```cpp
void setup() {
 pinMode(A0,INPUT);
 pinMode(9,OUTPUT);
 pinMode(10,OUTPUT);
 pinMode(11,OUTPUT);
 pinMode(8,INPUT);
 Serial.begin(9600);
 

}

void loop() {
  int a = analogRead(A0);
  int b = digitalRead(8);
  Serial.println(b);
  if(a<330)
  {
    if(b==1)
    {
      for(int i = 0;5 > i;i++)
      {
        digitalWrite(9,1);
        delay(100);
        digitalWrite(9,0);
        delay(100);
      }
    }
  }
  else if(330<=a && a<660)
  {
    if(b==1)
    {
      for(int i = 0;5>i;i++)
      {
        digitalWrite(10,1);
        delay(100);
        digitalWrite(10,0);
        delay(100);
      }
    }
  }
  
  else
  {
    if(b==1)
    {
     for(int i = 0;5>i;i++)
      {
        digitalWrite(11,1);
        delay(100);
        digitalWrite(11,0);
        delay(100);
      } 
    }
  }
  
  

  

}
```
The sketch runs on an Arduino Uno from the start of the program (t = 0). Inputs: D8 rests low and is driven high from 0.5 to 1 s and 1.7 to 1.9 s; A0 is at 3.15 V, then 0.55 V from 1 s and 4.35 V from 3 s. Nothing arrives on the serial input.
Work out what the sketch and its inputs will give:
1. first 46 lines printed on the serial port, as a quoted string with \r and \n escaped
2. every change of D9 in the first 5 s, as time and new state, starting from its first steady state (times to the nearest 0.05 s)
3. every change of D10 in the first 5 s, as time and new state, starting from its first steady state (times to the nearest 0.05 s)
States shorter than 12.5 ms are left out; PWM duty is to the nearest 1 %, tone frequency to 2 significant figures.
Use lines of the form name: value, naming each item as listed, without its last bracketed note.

first 46 lines printed on the serial port, as a quoted string with \r and \n escaped: "0\r\n0\r\n0\r\n0\r\n0\r\n0\r\n0\r\n0\r\n0\r\n0\r\n0\r\n0\r\n0\r\n0\r\n0\r\n0\r\n0\r\n0\r\n0\r\n0\r\n0\r\n0\r\n0\r\n0\r\n0\r\n0\r\n0\r\n0\r\n0\r\n0\r\n0\r\n0\r\n0\r\n0\r\n0\r\n0\r\n0\r\n0\r\n0\r\n0\r\n0\r\n0\r\n0\r\n0\r\n0\r\n0\r\n"
every change of D9 in the first 5 s, as time and new state, starting from its first steady state: 0 s low; 1.7 s high; 1.8 s low; 1.9 s high; 2 s low; 2.1 s high; 2.2 s low; 2.3 s high; 2.4 s low; 2.5 s high; 2.6 s low
every change of D10 in the first 5 s, as time and new state, starting from its first steady state: 0 s low; 0.5 s high; 0.6 s low; 0.7 s high; 0.8 s low; 0.9 s high; 1 s low; 1.1 s high; 1.2 s low; 1.3 s high; 1.4 s low
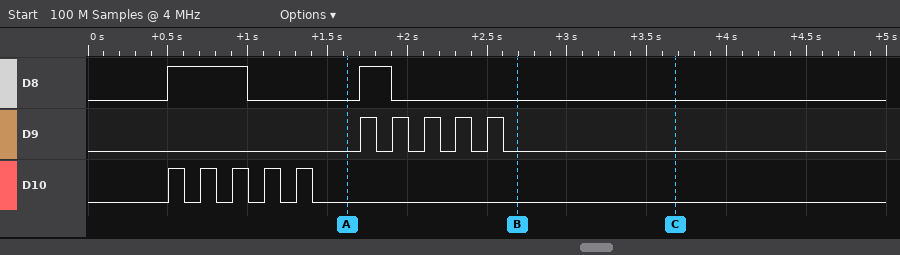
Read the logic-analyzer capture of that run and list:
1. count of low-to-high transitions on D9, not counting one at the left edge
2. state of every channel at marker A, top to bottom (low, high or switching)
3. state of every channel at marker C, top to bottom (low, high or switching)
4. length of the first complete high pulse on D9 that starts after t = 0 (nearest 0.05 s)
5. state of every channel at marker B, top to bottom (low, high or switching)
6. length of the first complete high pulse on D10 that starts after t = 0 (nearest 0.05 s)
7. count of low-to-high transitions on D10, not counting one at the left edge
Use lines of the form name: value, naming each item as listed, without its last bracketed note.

count of low-to-high transitions on D9, not counting one at the left edge: 5
state of every channel at marker A, top to bottom: D8 low, D9 low, D10 low
state of every channel at marker C, top to bottom: D8 low, D9 low, D10 low
length of the first complete high pulse on D9 that starts after t = 0: 0.10 s
state of every channel at marker B, top to bottom: D8 low, D9 low, D10 low
length of the first complete high pulse on D10 that starts after t = 0: 0.10 s
count of low-to-high transitions on D10, not counting one at the left edge: 5
